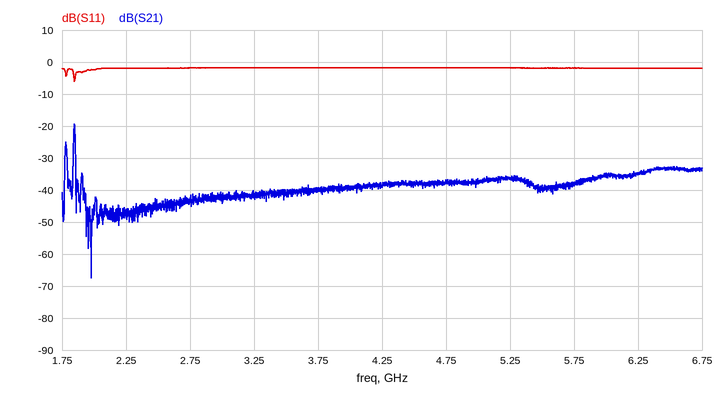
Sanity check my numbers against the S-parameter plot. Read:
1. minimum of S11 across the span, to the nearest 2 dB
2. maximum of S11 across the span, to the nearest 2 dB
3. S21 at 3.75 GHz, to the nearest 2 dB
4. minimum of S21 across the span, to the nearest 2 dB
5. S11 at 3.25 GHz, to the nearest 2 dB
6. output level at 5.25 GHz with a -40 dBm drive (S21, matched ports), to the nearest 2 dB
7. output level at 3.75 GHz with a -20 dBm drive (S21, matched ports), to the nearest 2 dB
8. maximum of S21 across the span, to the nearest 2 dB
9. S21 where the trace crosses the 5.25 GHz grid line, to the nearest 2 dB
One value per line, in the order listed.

-6 dB
-2 dB
-40 dB
-68 dB
-2 dB
-76 dBm
-60 dBm
-20 dB
-36 dB
